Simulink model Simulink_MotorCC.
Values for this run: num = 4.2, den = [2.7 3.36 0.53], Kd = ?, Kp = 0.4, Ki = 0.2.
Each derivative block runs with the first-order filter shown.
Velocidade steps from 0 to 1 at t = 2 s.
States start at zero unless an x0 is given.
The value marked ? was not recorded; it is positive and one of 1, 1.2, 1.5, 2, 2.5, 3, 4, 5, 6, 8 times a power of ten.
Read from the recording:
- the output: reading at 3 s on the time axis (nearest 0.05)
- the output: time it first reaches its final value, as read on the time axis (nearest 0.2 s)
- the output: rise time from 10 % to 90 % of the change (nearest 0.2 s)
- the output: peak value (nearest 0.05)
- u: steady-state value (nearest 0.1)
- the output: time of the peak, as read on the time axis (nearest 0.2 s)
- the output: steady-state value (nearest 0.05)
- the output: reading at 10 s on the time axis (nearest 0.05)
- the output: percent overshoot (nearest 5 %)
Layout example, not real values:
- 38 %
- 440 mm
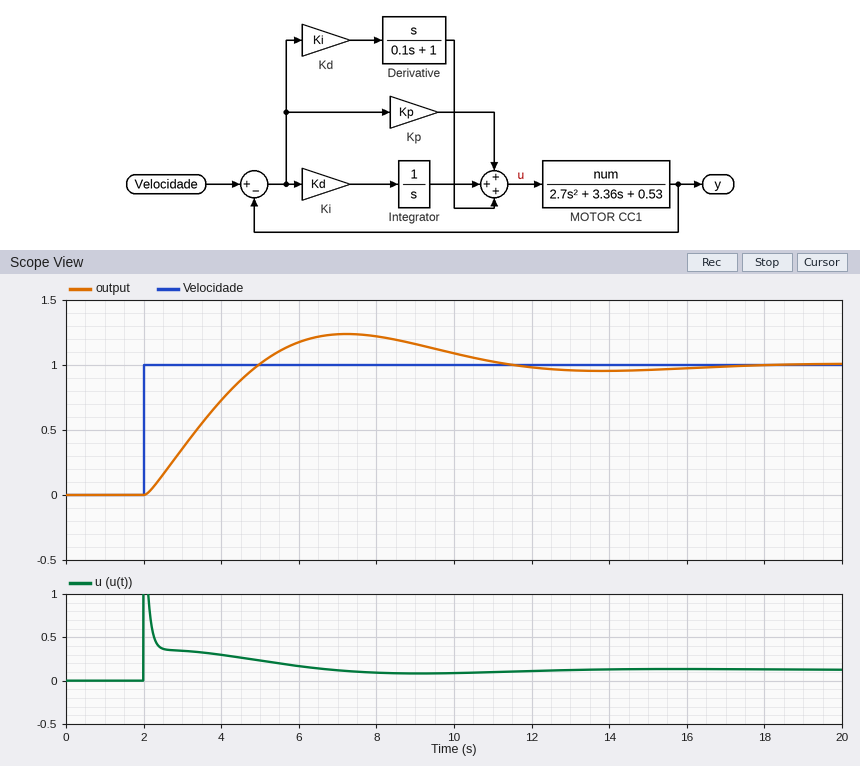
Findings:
- 0.35
- 5.0 s
- 2.2 s
- 1.25
- 0.1
- 7.2 s
- 1.00
- 1.10
- 25 %
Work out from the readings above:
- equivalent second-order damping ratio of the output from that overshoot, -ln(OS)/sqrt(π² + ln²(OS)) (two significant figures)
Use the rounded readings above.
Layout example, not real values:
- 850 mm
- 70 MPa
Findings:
- 0.40
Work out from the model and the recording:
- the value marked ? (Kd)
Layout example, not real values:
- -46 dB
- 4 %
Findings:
- 0.2
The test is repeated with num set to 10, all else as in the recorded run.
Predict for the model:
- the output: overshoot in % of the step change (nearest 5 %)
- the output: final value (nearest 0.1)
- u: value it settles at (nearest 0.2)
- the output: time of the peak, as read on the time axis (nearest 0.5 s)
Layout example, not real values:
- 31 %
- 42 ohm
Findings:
- 20 %
- 1.0
- 0.0
- 5.0 s
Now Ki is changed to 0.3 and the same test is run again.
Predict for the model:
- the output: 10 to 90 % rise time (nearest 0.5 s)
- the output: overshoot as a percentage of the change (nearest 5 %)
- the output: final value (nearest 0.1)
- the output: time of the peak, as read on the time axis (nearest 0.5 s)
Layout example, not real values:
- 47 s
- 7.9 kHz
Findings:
- 2.5 s
- 20 %
- 1.0
- 7.5 s
